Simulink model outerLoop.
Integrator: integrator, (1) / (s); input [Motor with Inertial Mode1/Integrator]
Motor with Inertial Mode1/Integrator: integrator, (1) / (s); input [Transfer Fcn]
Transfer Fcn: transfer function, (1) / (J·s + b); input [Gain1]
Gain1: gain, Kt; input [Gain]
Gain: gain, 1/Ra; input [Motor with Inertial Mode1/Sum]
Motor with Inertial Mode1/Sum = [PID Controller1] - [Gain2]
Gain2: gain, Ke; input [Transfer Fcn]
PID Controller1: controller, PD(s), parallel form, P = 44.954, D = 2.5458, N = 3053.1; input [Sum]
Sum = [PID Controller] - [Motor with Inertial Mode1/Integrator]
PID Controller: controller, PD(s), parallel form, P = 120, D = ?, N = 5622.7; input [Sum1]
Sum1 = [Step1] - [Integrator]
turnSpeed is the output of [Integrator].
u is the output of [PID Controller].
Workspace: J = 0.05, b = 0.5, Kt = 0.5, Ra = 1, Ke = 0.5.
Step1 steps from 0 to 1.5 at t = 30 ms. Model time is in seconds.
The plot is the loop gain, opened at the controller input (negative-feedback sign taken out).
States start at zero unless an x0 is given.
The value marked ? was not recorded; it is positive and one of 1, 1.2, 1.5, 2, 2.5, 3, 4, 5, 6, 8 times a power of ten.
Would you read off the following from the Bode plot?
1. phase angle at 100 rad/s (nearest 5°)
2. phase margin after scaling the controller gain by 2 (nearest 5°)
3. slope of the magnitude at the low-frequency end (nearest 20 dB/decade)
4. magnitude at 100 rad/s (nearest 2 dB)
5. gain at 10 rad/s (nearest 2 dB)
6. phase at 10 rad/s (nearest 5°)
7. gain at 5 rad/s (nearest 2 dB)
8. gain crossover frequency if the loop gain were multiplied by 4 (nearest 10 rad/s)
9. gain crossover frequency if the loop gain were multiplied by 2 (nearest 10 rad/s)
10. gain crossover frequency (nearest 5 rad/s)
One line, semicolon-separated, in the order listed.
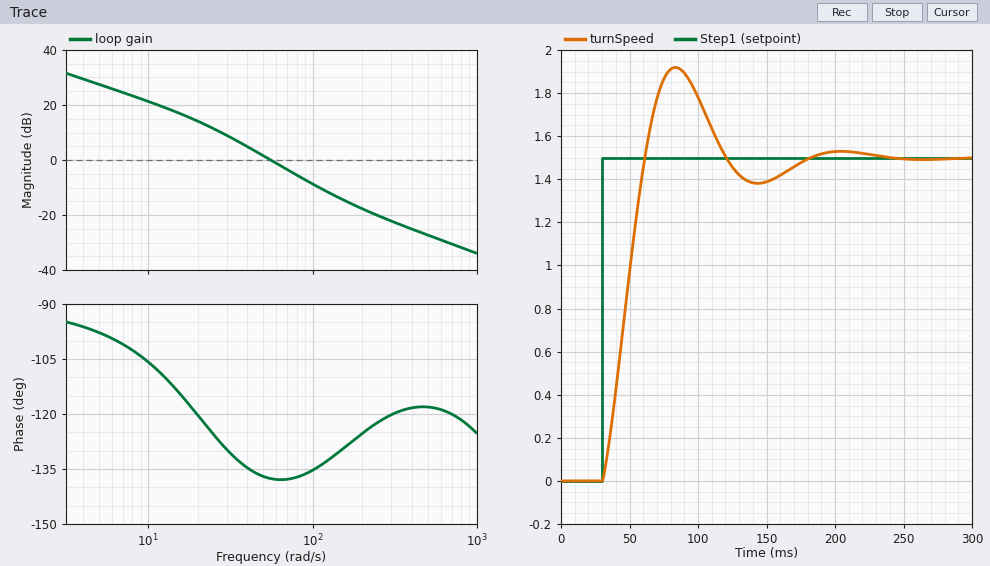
-135°; 45°; -20 dB/decade; -8 dB; 22 dB; -105°; 28 dB; 130 rad/s; 80 rad/s; 55 rad/s
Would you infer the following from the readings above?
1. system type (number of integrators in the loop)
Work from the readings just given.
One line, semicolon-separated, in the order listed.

1
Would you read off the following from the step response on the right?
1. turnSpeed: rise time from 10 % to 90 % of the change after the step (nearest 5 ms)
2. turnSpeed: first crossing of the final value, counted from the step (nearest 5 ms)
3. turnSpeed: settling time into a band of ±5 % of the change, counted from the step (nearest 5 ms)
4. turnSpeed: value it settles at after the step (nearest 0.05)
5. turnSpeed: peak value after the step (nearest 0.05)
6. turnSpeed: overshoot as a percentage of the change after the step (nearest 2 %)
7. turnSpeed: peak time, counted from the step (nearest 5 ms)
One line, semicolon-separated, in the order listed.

25 ms; 30 ms; 130 ms; 1.50; 1.90; 28 %; 55 ms
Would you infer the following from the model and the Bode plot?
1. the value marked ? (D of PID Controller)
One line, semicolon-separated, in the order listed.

0.8
